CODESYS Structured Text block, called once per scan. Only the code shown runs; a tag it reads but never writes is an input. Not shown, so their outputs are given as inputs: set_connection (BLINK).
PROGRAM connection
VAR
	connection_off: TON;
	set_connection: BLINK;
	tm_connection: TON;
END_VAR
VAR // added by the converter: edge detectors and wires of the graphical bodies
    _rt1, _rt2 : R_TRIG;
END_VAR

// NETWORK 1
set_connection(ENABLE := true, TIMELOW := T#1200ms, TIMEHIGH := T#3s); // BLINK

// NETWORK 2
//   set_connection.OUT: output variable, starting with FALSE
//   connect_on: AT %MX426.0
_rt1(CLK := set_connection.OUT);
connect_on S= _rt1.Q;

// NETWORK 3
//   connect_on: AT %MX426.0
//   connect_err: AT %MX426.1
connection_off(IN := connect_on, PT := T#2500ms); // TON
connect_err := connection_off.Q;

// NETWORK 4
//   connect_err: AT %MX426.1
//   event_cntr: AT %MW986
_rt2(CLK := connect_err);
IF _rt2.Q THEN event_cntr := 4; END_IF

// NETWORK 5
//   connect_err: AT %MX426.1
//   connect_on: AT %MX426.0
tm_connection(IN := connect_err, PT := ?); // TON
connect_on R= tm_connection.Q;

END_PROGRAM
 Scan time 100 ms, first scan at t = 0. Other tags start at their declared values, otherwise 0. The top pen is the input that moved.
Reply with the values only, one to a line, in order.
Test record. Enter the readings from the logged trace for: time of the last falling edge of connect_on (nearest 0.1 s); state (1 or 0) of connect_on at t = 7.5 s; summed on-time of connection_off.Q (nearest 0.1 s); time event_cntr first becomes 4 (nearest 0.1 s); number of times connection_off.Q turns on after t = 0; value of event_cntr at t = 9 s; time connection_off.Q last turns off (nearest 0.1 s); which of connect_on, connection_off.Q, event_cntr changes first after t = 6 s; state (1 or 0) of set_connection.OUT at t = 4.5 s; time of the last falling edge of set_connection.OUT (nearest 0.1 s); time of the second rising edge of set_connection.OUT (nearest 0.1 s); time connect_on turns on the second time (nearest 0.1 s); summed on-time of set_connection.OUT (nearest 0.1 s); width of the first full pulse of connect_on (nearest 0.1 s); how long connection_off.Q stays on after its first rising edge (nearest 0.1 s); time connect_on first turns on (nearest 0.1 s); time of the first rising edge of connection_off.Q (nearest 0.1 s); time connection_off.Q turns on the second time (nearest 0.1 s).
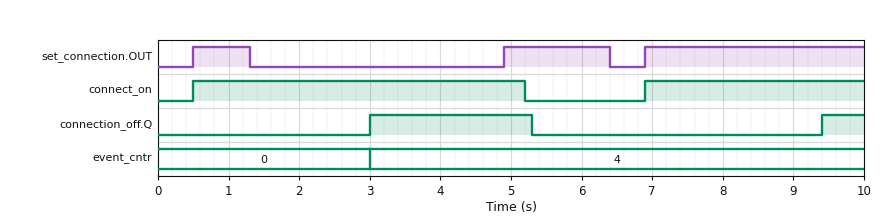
5.2 s
1
2.9 s
3.0 s
2
4
5.3 s
connect_on
0
6.4 s
4.9 s
6.9 s
5.4 s
4.7 s
2.3 s
0.5 s
3.0 s
9.4 s
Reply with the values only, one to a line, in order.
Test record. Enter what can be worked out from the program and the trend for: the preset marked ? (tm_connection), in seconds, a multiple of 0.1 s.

2.2 s
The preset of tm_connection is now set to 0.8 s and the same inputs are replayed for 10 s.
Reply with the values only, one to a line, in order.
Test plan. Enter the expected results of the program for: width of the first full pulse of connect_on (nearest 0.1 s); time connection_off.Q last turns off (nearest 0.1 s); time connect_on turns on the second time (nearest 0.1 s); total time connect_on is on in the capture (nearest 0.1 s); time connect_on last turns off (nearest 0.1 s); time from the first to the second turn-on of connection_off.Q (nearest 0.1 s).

3.3 s
8.3 s
4.9 s
6.6 s
8.2 s
4.4 s
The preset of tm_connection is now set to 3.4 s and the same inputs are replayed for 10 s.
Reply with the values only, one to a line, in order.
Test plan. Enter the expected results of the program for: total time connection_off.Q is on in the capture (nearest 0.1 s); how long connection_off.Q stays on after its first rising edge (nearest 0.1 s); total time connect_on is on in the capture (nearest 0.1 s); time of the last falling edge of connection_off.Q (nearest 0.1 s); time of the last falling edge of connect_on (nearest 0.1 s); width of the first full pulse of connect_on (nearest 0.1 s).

4.1 s
3.5 s
9.0 s
6.5 s
6.4 s
5.9 s
